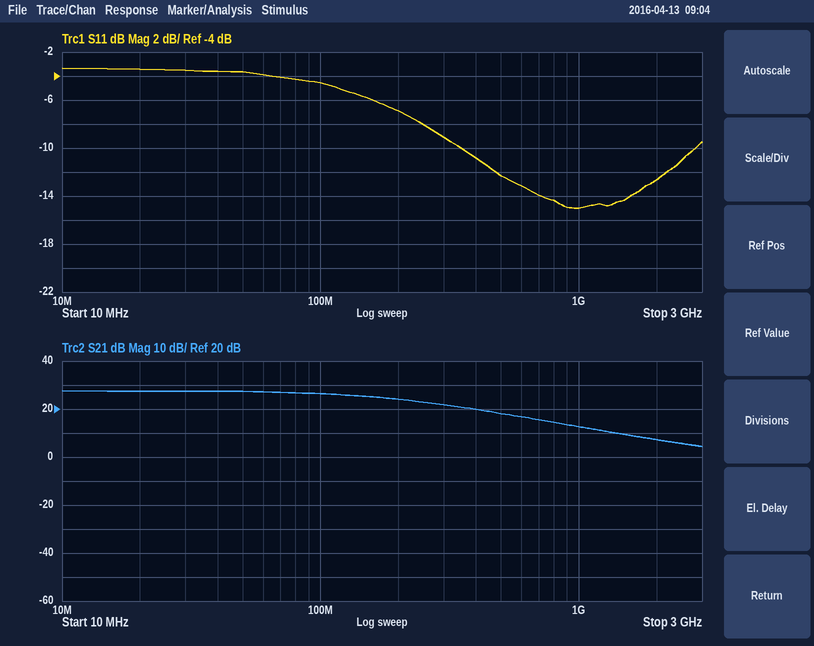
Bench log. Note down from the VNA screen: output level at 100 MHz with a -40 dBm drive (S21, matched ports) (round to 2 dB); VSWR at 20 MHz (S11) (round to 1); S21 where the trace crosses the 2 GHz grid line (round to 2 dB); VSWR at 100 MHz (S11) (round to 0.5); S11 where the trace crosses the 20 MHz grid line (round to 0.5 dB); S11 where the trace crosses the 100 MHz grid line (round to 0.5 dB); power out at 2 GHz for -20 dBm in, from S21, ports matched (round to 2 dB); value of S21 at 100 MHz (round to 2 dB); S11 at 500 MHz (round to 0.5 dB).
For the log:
-14 dBm
5
8 dB
4.0
-3.5 dB
-4.5 dB
-12 dBm
26 dB
-12.5 dB
